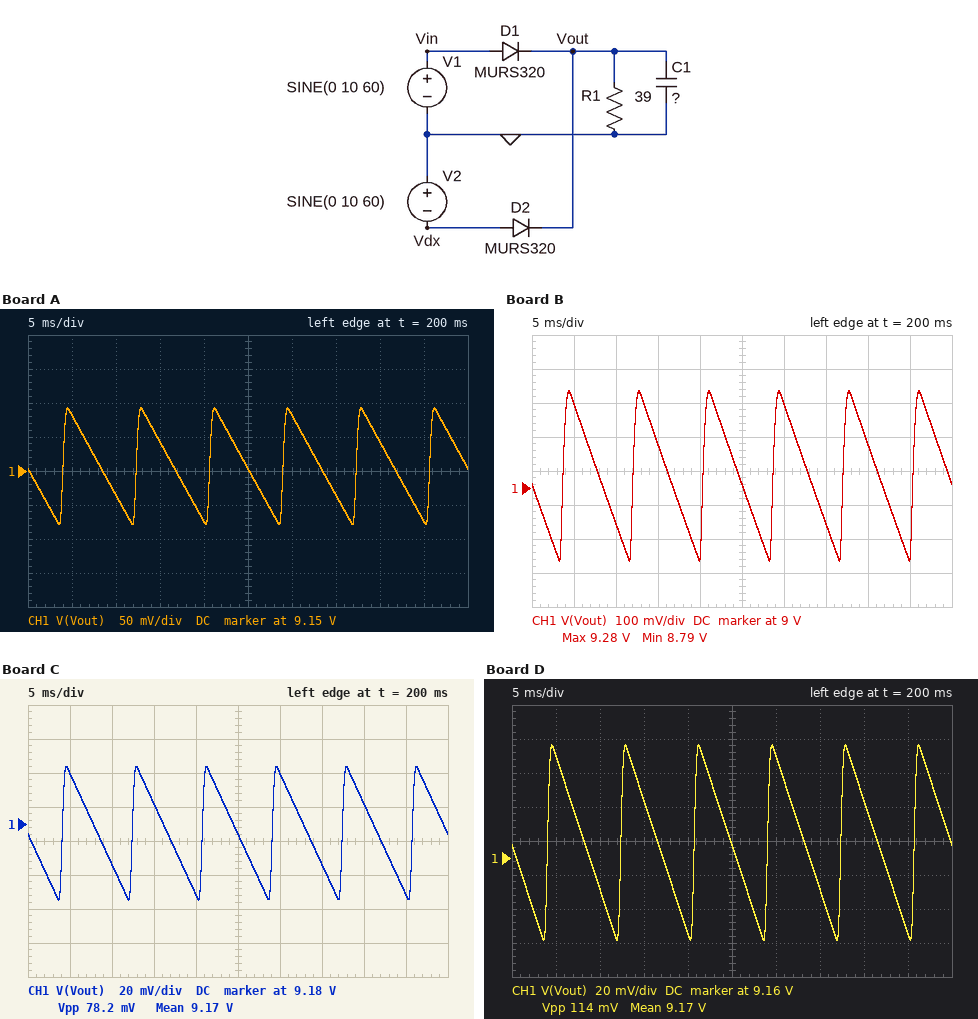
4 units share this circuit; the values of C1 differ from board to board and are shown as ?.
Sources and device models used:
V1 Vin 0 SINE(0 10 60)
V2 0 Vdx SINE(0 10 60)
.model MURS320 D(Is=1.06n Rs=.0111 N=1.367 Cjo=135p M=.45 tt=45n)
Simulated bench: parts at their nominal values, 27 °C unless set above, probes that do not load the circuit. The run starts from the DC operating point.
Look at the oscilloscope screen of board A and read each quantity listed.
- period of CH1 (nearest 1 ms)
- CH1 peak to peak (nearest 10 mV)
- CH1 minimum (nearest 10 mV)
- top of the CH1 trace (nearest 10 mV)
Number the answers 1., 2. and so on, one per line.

1. 8 ms
2. 170 mV
3. 9.07 V
4. 9.24 V
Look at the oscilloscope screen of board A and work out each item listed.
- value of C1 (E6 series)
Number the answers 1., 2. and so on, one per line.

1. 10 mF
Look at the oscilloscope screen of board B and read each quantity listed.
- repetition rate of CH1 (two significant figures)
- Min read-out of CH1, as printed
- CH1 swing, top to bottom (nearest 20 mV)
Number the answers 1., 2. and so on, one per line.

1. 120 Hz
2. 8.79 V
3. 500 mV
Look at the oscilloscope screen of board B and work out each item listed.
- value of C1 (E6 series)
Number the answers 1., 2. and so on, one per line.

1. 3.3 mF
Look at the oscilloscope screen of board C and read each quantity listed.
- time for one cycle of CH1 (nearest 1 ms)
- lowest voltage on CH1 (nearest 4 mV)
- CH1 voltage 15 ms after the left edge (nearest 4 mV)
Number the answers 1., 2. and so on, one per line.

1. 8 ms
2. 9.136 V
3. 9.192 V
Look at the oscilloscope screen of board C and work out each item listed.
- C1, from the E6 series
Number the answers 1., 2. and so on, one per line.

1. 22 mF
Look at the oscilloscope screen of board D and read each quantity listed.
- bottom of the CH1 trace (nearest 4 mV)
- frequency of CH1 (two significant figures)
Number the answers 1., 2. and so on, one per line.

1. 9.112 V
2. 120 Hz
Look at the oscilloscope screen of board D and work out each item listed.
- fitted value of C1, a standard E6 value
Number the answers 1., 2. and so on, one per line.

1. 15 mF
